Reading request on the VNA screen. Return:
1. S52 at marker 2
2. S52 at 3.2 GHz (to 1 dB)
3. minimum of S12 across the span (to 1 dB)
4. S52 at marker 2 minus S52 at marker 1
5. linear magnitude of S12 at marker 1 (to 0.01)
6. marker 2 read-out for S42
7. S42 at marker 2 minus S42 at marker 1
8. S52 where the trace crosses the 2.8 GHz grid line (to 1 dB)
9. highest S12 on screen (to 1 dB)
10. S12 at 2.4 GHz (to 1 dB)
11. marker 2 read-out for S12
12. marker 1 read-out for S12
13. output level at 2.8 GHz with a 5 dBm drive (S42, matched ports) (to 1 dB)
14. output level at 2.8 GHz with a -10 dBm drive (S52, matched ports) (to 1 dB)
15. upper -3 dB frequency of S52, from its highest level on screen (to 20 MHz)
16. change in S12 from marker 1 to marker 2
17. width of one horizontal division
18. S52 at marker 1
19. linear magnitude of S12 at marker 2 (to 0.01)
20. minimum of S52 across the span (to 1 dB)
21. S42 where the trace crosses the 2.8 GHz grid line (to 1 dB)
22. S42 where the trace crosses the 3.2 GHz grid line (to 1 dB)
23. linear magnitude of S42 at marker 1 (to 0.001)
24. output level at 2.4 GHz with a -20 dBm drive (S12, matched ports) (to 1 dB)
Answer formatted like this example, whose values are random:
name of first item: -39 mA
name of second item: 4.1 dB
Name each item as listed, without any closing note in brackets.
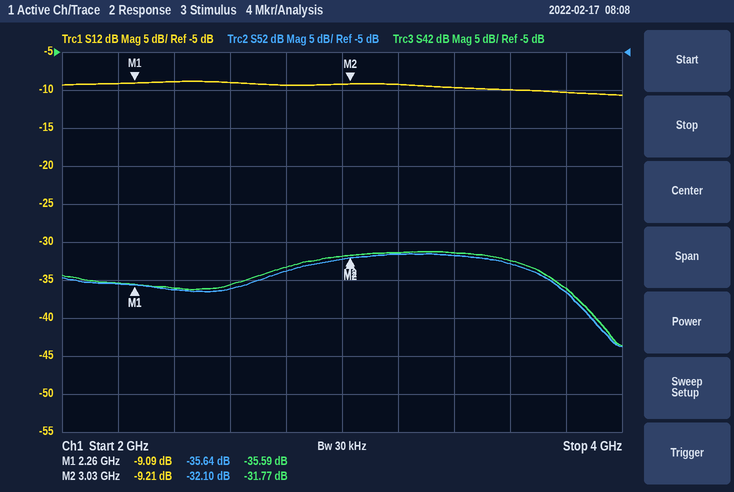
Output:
S52 at marker 2: -32.10 dB
S52 at 3.2 GHz: -32 dB
minimum of S12 across the span: -11 dB
S52 at marker 2 minus S52 at marker 1: 3.54 dB
linear magnitude of S12 at marker 1: 0.35
marker 2 read-out for S42: -31.77 dB
S42 at marker 2 minus S42 at marker 1: 3.82 dB
S52 where the trace crosses the 2.8 GHz grid line: -34 dB
highest S12 on screen: -9 dB
S12 at 2.4 GHz: -9 dB
marker 2 read-out for S12: -9.21 dB
marker 1 read-out for S12: -9.09 dB
output level at 2.8 GHz with a 5 dBm drive (S42, matched ports): -28 dBm
output level at 2.8 GHz with a -10 dBm drive (S52, matched ports): -44 dBm
upper -3 dB frequency of S52, from its highest level on screen: 3.72 GHz
change in S12 from marker 1 to marker 2: -0.12 dB
width of one horizontal division: 200 MHz
S52 at marker 1: -35.64 dB
linear magnitude of S12 at marker 2: 0.35
minimum of S52 across the span: -44 dB
S42 where the trace crosses the 2.8 GHz grid line: -33 dB
S42 where the trace crosses the 3.2 GHz grid line: -31 dB
linear magnitude of S42 at marker 1: 0.017
output level at 2.4 GHz with a -20 dBm drive (S12, matched ports): -29 dBm
